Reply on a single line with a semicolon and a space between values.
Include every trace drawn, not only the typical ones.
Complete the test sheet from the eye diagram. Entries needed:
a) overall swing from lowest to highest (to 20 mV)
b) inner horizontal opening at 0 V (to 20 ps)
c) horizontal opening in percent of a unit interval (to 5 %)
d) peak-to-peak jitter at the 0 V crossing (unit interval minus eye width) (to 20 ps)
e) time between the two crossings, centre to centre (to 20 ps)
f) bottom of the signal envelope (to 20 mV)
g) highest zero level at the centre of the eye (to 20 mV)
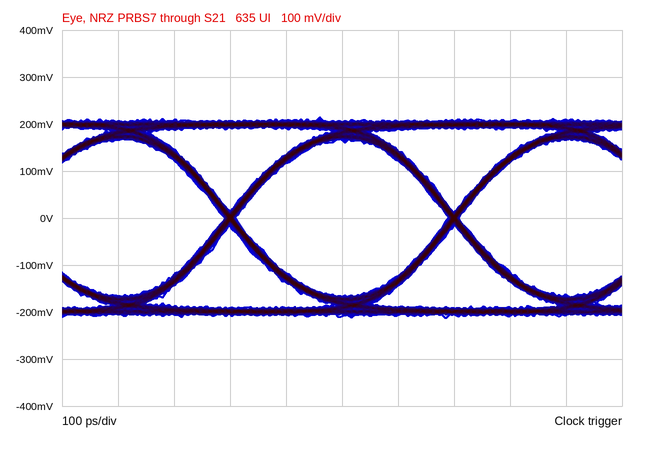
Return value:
420 mV; 380 ps; 95 %; 20 ps; 400 ps; -220 mV; -160 mV
